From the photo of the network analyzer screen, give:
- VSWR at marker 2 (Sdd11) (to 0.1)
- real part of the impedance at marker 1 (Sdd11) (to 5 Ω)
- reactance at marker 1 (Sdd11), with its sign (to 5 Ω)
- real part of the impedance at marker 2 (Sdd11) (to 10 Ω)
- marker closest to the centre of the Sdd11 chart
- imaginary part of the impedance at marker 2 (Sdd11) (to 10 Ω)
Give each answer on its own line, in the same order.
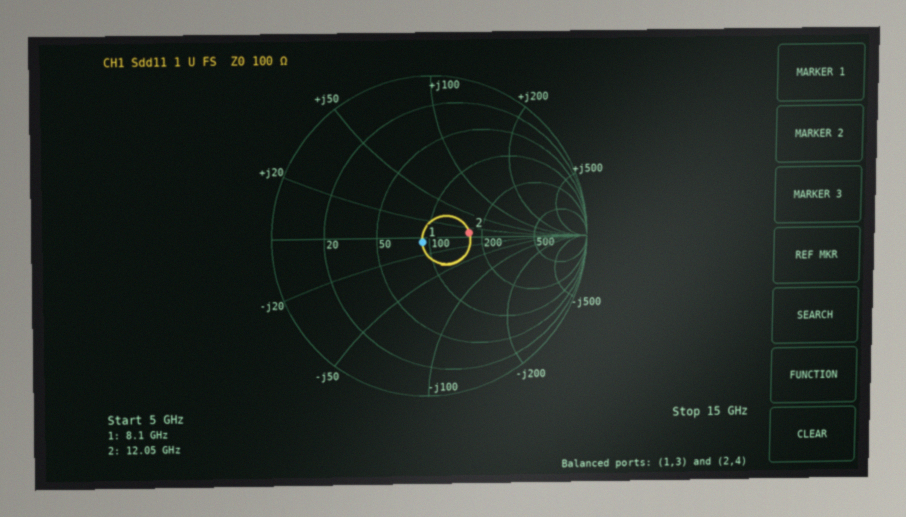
1.7
90 Ω
-5 Ω
170 Ω
marker 1
+10 Ω
